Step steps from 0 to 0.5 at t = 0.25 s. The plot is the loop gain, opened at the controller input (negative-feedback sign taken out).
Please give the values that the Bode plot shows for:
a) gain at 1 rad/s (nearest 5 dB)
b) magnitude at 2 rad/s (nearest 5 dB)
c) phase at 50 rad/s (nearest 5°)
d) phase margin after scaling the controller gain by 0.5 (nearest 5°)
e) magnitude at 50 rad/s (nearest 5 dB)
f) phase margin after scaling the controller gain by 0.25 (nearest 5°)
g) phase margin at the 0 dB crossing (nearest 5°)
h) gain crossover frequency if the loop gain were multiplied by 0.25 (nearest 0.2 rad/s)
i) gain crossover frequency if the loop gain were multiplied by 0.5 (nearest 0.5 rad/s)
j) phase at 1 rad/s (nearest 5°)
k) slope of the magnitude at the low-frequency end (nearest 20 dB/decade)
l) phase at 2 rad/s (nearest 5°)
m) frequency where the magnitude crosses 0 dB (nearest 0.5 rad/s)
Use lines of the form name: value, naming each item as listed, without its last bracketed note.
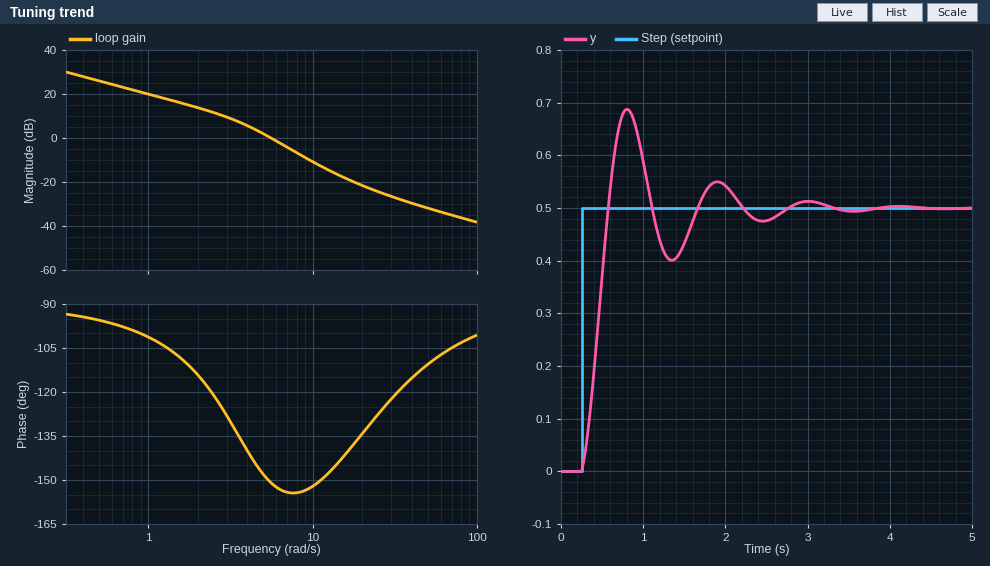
gain at 1 rad/s: 20 dB
magnitude at 2 rad/s: 15 dB
phase at 50 rad/s: -110°
phase margin after scaling the controller gain by 0.5: 40°
magnitude at 50 rad/s: -30 dB
phase margin after scaling the controller gain by 0.25: 60°
phase margin at the 0 dB crossing: 30°
gain crossover frequency if the loop gain were multiplied by 0.25: 2.4 rad/s
gain crossover frequency if the loop gain were multiplied by 0.5: 4.0 rad/s
phase at 1 rad/s: -100°
slope of the magnitude at the low-frequency end: -20 dB/decade
phase at 2 rad/s: -115°
frequency where the magnitude crosses 0 dB: 5.5 rad/s
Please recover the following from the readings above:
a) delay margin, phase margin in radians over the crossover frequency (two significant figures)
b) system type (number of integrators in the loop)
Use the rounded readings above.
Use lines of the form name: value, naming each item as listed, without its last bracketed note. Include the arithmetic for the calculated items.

delay margin, phase margin in radians over the crossover frequency: 30 × π / 180 / 5.5 = 0.095 s
system type: 1
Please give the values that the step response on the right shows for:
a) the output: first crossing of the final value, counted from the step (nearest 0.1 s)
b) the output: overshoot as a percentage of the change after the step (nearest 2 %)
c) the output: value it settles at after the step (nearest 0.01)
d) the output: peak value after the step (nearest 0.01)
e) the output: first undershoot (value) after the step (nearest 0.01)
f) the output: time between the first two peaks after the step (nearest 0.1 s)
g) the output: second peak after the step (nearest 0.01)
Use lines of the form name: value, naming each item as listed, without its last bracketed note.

the output: first crossing of the final value, counted from the step: 0.3 s
the output: overshoot as a percentage of the change after the step: 38 %
the output: value it settles at after the step: 0.50
the output: peak value after the step: 0.69
the output: first undershoot (value) after the step: 0.40
the output: time between the first two peaks after the step: 1.1 s
the output: second peak after the step: 0.55
